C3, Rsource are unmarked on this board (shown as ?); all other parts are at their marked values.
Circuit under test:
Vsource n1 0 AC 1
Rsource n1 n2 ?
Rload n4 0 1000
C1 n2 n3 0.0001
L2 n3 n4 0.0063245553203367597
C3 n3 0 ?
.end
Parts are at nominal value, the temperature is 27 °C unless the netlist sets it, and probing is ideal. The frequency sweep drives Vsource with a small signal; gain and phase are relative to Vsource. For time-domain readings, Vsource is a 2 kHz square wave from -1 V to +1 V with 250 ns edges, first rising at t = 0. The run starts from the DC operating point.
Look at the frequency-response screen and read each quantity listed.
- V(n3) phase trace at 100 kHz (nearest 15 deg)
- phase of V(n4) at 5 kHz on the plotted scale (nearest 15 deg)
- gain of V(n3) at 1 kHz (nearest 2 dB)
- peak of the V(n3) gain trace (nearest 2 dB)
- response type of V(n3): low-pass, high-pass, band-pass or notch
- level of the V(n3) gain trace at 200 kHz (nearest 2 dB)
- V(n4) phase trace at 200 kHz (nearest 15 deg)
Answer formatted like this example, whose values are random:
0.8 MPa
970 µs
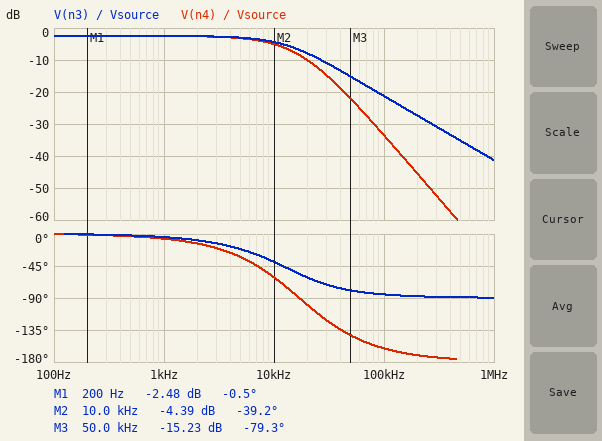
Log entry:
-90 deg
-30 deg
-2 dB
-2 dB
low-pass
-28 dB
-165 deg
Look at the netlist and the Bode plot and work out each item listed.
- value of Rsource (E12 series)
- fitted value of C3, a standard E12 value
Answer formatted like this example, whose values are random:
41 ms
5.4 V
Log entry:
330 Ω
56 nF
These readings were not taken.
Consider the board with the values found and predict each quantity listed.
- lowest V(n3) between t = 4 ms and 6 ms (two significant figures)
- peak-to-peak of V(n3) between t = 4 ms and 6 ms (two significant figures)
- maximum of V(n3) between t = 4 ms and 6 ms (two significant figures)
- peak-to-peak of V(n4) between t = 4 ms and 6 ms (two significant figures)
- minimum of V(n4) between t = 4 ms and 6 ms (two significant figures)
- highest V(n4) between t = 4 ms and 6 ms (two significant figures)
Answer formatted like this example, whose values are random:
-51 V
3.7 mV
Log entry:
-33 mV
1.5 V
1.5 V
1.5 V
-33 mV
1.5 V
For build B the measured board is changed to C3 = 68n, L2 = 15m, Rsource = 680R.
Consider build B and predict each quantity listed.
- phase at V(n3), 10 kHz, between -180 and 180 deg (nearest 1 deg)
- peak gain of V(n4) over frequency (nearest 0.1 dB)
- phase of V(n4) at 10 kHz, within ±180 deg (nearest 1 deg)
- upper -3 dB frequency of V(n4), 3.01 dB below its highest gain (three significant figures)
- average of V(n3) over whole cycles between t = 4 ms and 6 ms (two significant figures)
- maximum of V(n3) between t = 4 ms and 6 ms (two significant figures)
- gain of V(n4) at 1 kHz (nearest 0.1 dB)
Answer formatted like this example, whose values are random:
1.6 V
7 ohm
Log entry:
-62 deg
-4.5 dB
-105 deg
5.87 kHz
580 mV
1.2 V
-4.6 dB
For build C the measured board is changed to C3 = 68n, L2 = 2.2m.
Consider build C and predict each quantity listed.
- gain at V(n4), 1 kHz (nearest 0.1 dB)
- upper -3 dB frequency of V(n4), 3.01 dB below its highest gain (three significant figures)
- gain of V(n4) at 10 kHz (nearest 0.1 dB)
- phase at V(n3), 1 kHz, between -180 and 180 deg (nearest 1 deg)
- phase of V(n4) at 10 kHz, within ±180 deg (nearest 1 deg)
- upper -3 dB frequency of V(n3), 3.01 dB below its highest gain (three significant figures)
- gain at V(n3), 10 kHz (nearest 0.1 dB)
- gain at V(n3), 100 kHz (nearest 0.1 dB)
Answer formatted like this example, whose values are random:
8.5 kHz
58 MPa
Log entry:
-2.5 dB
9.62 kHz
-5.7 dB
-6 deg
-54 deg
9.79 kHz
-5.6 dB
-22.9 dB
